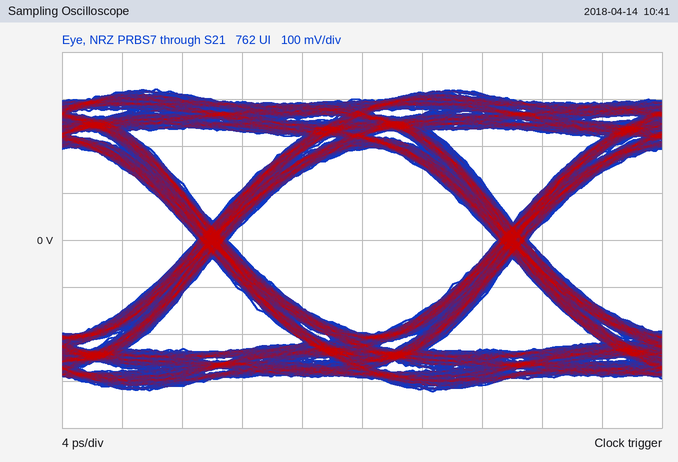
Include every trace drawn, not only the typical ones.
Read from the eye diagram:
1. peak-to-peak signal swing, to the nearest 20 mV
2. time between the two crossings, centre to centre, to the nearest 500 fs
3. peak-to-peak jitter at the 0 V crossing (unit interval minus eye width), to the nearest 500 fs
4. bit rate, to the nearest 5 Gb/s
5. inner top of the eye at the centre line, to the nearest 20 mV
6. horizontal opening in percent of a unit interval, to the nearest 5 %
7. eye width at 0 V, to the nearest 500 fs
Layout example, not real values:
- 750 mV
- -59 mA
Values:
- 640 mV
- 20.0 ps
- 2.0 ps
- 50 Gb/s
- 200 mV
- 90 %
- 18.0 ps
